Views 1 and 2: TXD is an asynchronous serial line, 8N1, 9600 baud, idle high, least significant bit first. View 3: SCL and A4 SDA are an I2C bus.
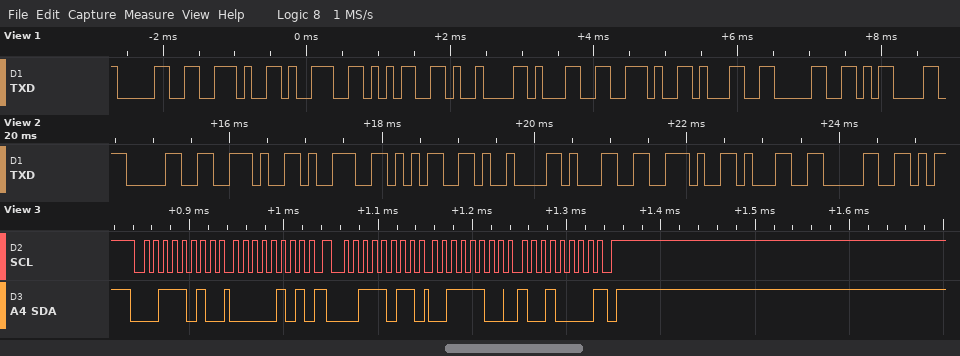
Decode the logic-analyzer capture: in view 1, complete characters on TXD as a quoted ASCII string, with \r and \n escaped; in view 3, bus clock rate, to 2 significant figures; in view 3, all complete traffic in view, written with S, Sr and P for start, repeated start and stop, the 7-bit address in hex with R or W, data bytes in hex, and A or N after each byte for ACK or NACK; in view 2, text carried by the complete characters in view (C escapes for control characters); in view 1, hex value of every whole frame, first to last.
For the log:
"0.95\t1.10\r"
100 kHz
S 1DW A 05 A Sr 1DR A 3C A 90 N P
"0.95\t1.10"
30 2E 39 35 09 31 2E 31 30 0D
